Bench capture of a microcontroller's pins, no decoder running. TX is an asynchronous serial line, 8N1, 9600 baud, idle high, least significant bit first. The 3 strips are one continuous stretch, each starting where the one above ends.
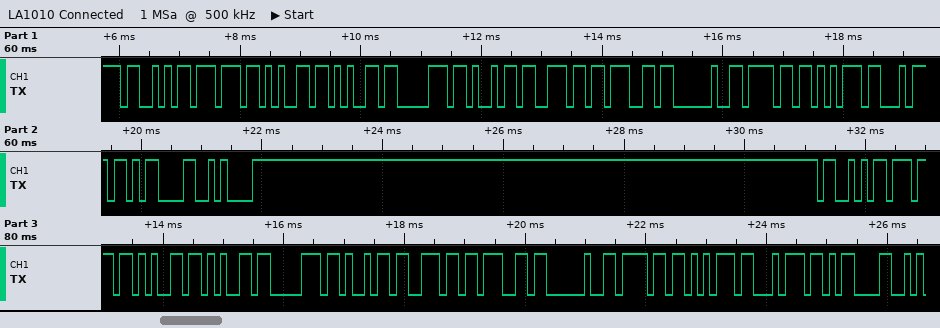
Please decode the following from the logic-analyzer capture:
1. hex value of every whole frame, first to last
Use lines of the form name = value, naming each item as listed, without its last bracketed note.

hex value of every whole frame, first to last = 53 77 65 65 70 69 6E 67 20 6F 75 74 0D 0A 53 77 65 65 70 69 6E 67 20 6F 75 74 0D
